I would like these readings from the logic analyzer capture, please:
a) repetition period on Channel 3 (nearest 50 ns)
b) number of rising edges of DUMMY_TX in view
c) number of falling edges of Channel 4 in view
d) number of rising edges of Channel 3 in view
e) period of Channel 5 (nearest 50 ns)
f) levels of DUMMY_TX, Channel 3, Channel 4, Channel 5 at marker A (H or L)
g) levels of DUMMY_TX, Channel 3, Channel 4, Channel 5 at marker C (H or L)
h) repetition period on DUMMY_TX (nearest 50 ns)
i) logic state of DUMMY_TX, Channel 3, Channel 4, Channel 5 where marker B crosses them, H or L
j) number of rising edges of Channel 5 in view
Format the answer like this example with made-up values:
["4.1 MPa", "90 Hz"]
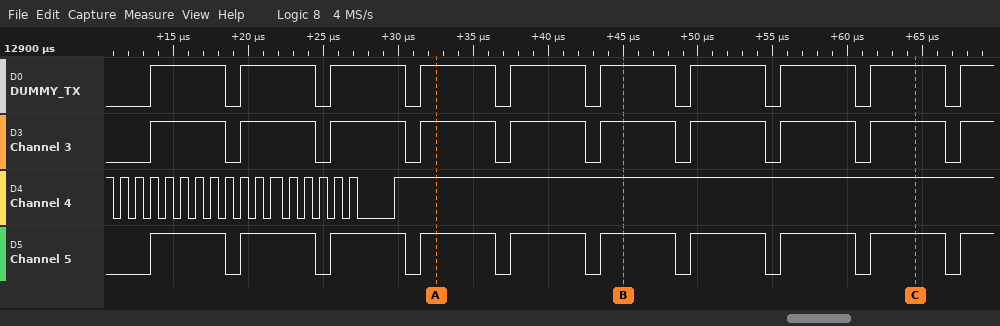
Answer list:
["6000 ns", "10", "17", "10", "6000 ns", "DUMMY_TX=H, Channel 3=H, Channel 4=H, Channel 5=H", "DUMMY_TX=H, Channel 3=H, Channel 4=H, Channel 5=H", "6000 ns", "DUMMY_TX=H, Channel 3=H, Channel 4=H, Channel 5=H", "10"]
